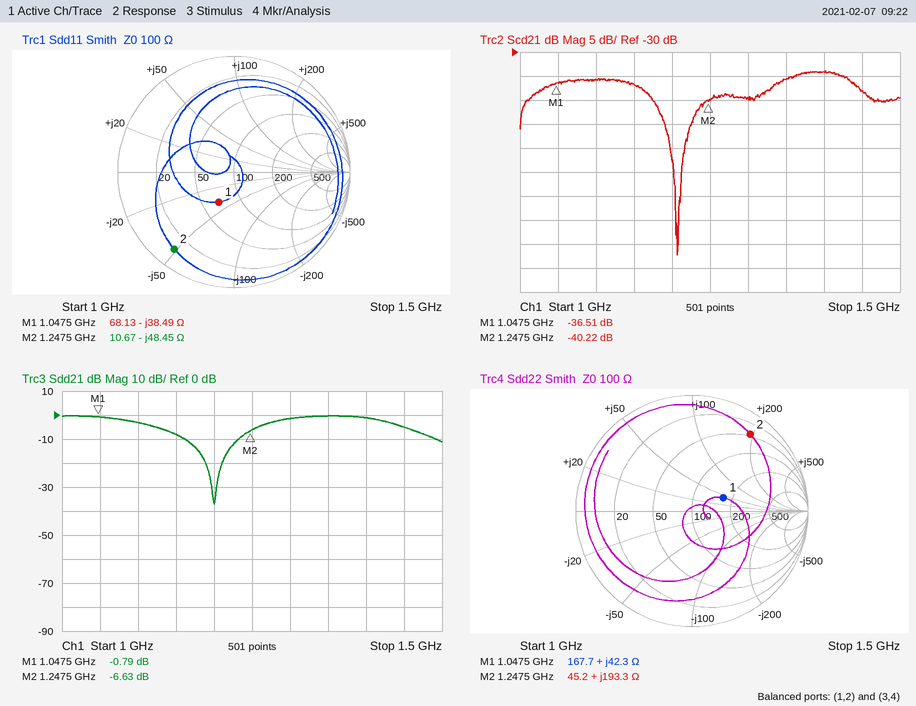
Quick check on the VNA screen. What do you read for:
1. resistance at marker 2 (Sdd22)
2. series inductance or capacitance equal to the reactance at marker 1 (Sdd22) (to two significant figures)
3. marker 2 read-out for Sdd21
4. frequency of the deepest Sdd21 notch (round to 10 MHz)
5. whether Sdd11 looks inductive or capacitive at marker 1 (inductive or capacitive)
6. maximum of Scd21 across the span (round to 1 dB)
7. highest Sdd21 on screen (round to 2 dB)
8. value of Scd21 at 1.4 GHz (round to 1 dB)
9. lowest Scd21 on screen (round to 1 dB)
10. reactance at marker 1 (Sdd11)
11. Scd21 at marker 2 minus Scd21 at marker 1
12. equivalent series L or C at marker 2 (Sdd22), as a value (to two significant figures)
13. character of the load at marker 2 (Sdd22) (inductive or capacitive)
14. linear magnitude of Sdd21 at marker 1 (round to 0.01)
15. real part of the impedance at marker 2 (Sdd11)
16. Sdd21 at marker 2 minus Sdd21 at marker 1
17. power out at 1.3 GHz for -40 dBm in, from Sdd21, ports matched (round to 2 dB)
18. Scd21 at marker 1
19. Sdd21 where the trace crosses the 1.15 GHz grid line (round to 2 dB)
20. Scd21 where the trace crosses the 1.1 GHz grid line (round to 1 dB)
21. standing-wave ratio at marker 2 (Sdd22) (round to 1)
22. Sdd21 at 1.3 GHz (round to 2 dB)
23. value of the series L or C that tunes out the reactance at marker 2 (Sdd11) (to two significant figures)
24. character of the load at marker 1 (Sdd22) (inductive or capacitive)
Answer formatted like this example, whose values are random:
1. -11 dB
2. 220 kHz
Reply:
1. 45.2 Ω
2. 6.4 nH
3. -6.63 dB
4. 1.20 GHz
5. capacitive
6. -34 dB
7. 0 dB
8. -34 dB
9. -72 dB
10. -38.49 Ω
11. -3.71 dB
12. 25 nH
13. inductive
14. 0.91
15. 10.67 Ω
16. -5.84 dB
17. -42 dBm
18. -36.51 dB
19. -8 dB
20. -36 dB
21. 11
22. -2 dB
23. 6.2 nH
24. inductive
